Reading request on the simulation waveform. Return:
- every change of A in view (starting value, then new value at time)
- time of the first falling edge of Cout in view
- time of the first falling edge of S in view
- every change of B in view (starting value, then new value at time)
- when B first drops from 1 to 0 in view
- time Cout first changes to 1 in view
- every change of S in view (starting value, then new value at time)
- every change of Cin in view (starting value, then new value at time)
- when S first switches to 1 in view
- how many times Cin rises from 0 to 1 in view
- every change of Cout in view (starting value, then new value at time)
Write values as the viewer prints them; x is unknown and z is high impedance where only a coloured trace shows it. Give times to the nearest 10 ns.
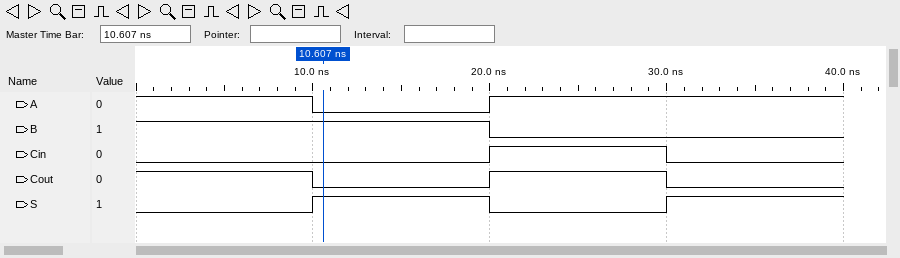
1, 0 at 10 ns, 1 at 20 ns
10 ns
20 ns
1, 0 at 20 ns
20 ns
20 ns
0, 1 at 10 ns, 0 at 20 ns, 1 at 30 ns
0, 1 at 20 ns, 0 at 30 ns
10 ns
1
1, 0 at 10 ns, 1 at 20 ns, 0 at 30 ns
